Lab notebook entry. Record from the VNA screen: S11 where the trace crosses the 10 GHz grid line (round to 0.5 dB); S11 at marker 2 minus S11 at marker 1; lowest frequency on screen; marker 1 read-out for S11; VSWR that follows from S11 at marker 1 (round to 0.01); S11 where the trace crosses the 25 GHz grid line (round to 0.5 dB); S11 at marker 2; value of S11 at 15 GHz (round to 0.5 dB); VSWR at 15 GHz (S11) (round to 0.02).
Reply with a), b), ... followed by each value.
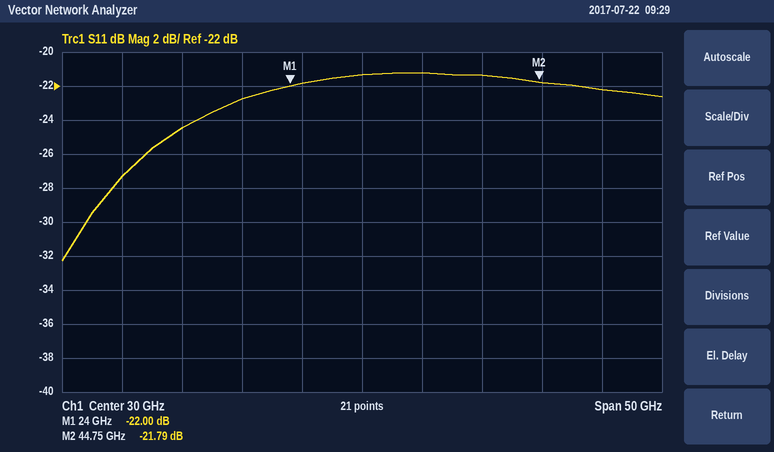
a) -27.5 dB
b) 0.21 dB
c) 5 GHz
d) -22.00 dB
e) 1.17
f) -22.0 dB
g) -21.79 dB
h) -24.5 dB
i) 1.12
